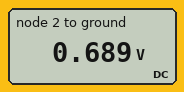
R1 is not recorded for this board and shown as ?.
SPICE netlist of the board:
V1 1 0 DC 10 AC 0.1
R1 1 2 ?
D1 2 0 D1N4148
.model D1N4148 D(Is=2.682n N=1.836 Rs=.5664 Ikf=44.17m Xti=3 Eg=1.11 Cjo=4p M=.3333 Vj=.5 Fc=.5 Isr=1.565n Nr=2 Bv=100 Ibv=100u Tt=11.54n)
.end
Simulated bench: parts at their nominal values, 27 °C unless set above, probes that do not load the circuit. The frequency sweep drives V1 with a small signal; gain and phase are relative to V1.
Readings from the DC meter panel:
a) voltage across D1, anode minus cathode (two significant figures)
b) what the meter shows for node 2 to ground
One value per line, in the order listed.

690 mV
0.689 V
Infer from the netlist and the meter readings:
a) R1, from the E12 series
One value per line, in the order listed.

2.2 kΩ
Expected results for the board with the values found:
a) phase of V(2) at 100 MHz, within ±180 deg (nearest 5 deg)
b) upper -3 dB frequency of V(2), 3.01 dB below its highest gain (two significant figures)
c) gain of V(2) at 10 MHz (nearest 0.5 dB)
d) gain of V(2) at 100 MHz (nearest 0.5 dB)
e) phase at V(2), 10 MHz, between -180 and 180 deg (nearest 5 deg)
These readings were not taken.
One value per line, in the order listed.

-65 deg
14 MHz
-46.0 dB
-61.0 dB
-35 deg
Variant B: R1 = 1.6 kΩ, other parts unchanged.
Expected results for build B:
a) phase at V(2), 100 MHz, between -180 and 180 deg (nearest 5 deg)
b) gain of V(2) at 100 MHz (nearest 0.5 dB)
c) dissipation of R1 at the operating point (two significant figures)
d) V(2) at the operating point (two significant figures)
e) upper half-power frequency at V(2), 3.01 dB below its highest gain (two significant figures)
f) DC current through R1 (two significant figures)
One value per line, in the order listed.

-60 deg
-60.5 dB
54 mW
710 mV
14 MHz
5.8 mA
